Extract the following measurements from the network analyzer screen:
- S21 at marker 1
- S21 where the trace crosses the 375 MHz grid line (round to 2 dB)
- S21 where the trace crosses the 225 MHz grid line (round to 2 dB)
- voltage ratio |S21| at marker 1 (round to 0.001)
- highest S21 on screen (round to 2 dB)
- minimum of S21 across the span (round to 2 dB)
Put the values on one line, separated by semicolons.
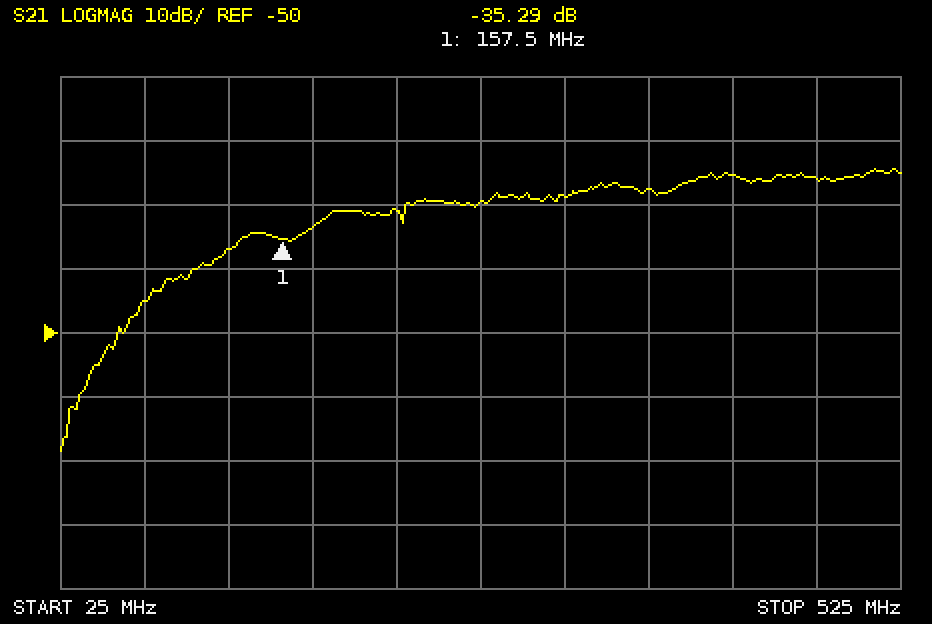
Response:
-35.29 dB; -28 dB; -30 dB; 0.017; -24 dB; -68 dB
